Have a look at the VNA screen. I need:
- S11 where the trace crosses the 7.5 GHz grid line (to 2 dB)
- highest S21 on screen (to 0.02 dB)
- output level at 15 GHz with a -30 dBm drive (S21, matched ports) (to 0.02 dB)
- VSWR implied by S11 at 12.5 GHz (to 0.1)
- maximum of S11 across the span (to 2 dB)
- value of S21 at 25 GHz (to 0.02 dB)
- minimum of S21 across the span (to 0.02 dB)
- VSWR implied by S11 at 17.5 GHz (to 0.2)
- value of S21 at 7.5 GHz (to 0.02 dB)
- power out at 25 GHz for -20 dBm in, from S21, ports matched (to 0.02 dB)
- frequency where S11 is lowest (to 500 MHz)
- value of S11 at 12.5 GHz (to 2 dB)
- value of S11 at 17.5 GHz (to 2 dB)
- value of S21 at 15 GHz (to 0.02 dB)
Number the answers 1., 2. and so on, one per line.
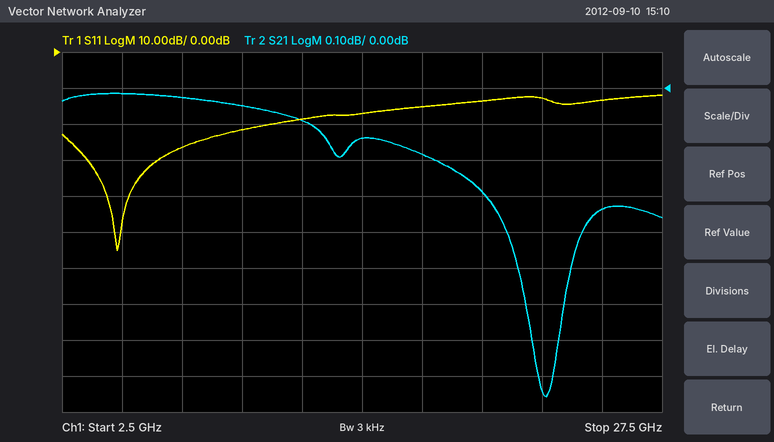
1. -26 dB
2. -0.02 dB
3. -30.14 dBm
4. 1.3
5. -12 dB
6. -0.34 dB
7. -0.86 dB
8. 1.4
9. -0.02 dB
10. -20.34 dBm
11. 5.0 GHz
12. -18 dB
13. -16 dB
14. -0.14 dB
